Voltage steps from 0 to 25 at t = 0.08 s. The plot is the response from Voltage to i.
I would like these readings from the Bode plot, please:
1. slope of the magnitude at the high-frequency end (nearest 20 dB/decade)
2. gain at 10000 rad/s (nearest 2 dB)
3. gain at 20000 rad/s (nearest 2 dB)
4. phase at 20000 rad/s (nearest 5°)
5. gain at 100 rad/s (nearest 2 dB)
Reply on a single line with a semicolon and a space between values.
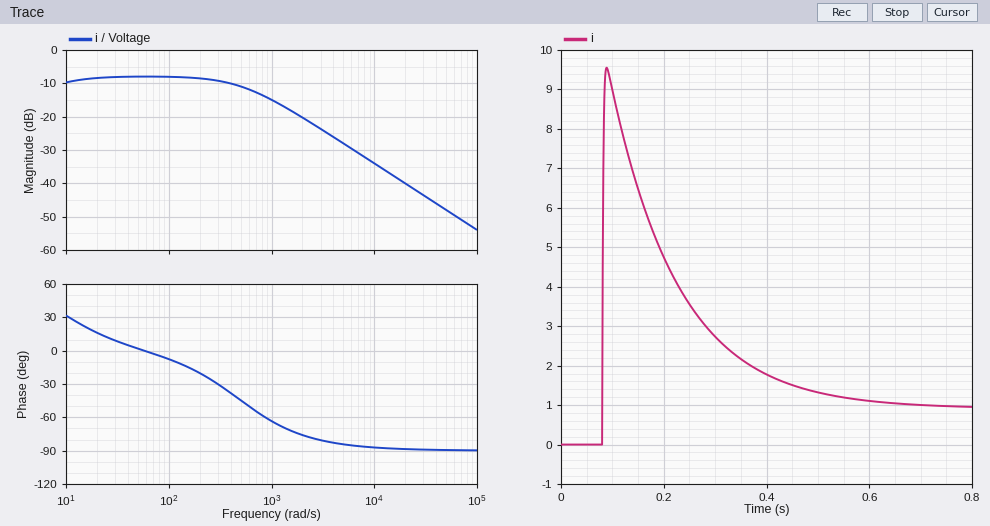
-20 dB/decade; -34 dB; -40 dB; -90°; -8 dB
